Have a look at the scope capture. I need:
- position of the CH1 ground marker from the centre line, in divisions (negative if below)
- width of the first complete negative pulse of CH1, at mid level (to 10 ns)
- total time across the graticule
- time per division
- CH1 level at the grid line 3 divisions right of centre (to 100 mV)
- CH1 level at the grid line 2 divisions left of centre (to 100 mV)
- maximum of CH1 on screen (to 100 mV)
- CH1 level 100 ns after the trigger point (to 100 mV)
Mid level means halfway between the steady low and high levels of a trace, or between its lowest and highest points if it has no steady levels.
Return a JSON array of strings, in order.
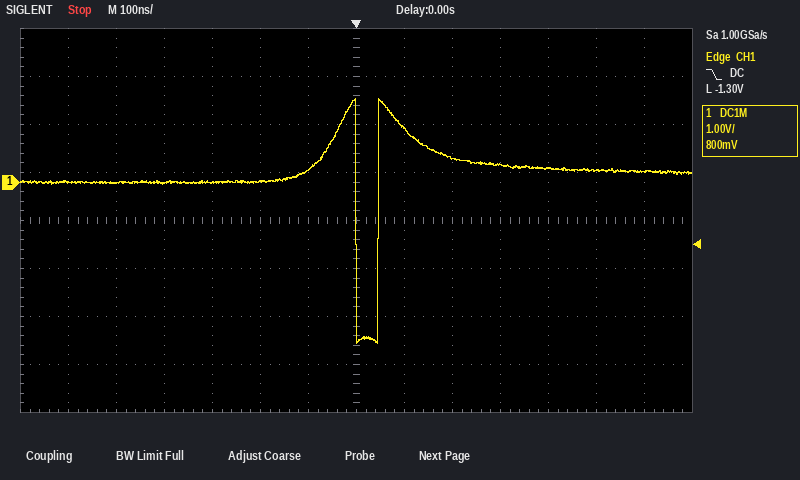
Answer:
["+0.8 div", "50 ns", "1.4 µs", "100 ns", "400 mV", "0.0 V", "1.7 V", "1.1 V"]
